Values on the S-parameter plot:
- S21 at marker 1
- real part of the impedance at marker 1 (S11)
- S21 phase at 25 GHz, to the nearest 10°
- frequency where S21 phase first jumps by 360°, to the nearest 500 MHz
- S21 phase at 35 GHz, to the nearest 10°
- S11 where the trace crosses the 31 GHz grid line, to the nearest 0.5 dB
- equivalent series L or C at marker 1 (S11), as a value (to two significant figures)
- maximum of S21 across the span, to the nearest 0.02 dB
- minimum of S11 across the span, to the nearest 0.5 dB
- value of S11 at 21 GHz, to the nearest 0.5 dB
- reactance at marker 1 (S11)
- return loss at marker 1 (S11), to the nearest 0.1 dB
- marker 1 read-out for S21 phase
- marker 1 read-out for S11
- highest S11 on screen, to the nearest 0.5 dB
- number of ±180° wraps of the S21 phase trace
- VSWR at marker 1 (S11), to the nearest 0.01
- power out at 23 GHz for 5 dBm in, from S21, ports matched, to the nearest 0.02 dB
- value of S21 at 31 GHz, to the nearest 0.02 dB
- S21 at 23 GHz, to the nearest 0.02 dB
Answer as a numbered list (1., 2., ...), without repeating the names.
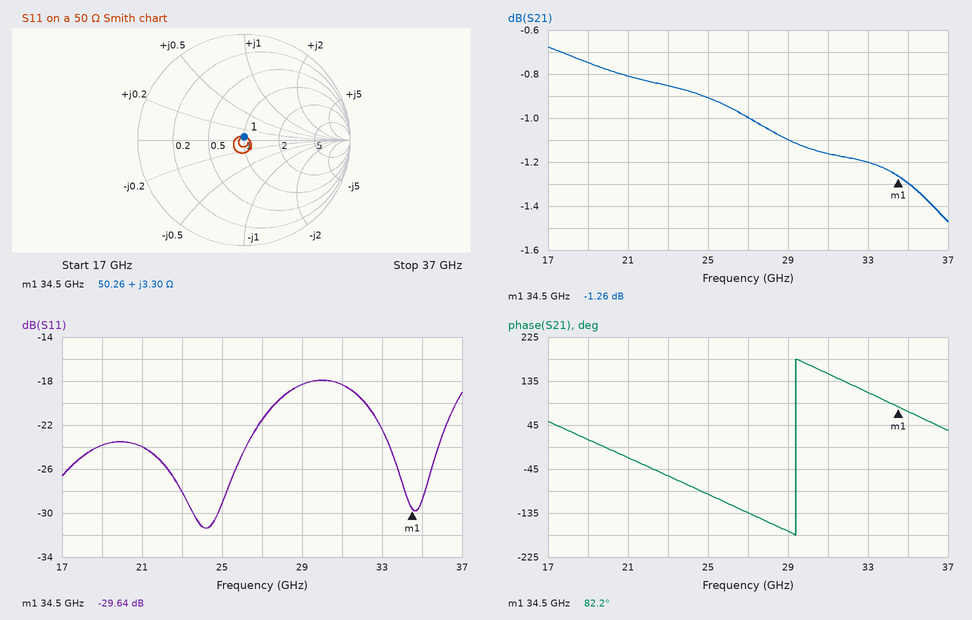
1. -1.26 dB
2. 50.26 Ω
3. -100°
4. 29.5 GHz
5. 70°
6. -18.5 dB
7. 15 pH
8. -0.68 dB
9. -31.5 dB
10. -24.0 dB
11. +3.30 Ω
12. 29.6 dB
13. 82.2°
14. -29.64 dB
15. -18.0 dB
16. 1
17. 1.07
18. 4.14 dBm
19. -1.16 dB
20. -0.86 dB
